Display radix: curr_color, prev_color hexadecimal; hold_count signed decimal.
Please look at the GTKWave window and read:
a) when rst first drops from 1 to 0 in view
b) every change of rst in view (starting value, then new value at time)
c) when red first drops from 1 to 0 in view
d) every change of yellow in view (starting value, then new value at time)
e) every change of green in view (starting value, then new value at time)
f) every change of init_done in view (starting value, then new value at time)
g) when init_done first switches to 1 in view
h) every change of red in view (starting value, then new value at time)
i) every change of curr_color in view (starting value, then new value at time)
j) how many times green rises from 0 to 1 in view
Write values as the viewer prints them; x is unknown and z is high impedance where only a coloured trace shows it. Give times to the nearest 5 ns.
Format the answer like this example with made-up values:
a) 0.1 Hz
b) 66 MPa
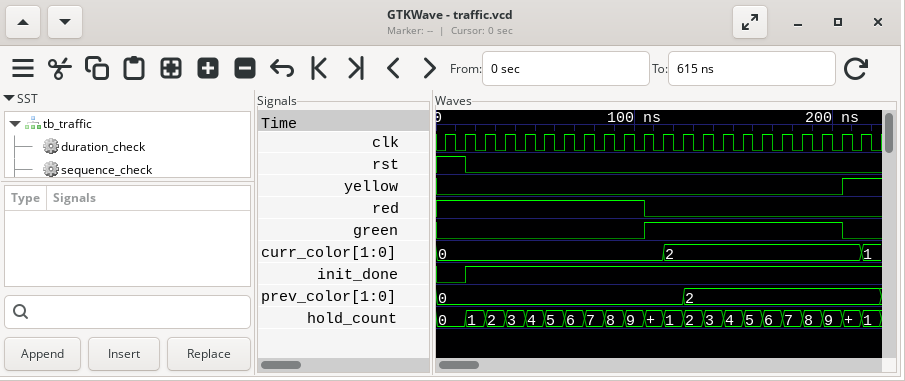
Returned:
a) 15 ns
b) 1, 0 at 15 ns
c) 105 ns
d) 0, 1 at 205 ns
e) 0, 1 at 105 ns, 0 at 205 ns
f) 0, 1 at 15 ns
g) 15 ns
h) 1, 0 at 105 ns
i) 0, 2 at 115 ns, 1 at 215 ns
j) 1
